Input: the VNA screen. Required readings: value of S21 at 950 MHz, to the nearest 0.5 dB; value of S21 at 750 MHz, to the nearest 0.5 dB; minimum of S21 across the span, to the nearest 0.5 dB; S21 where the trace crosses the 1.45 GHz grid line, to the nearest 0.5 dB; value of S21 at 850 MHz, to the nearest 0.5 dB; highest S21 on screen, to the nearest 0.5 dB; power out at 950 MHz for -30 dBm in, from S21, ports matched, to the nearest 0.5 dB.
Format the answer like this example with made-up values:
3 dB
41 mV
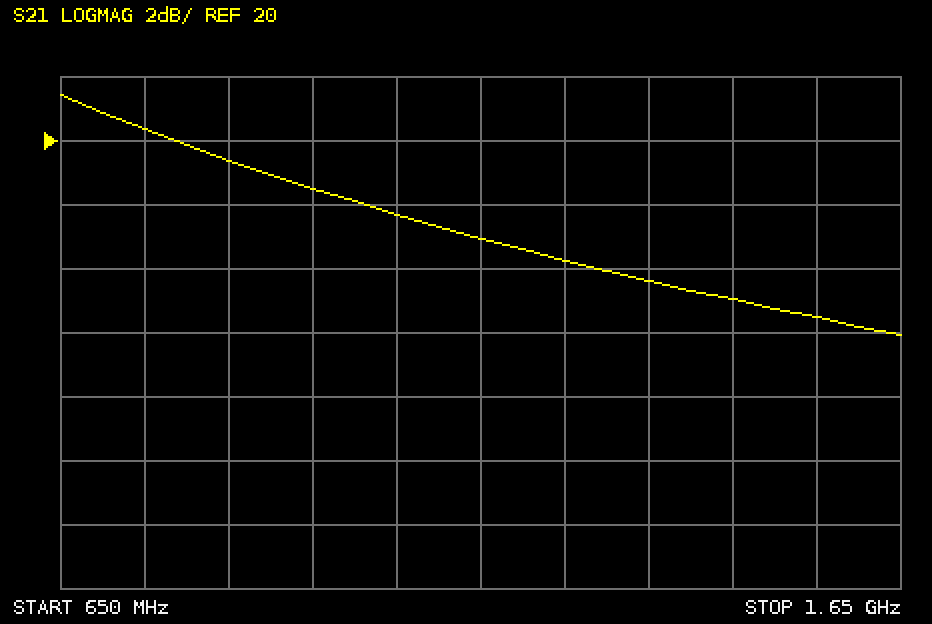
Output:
18.5 dB
20.5 dB
14.0 dB
15.0 dB
19.5 dB
21.5 dB
-11.5 dBm
